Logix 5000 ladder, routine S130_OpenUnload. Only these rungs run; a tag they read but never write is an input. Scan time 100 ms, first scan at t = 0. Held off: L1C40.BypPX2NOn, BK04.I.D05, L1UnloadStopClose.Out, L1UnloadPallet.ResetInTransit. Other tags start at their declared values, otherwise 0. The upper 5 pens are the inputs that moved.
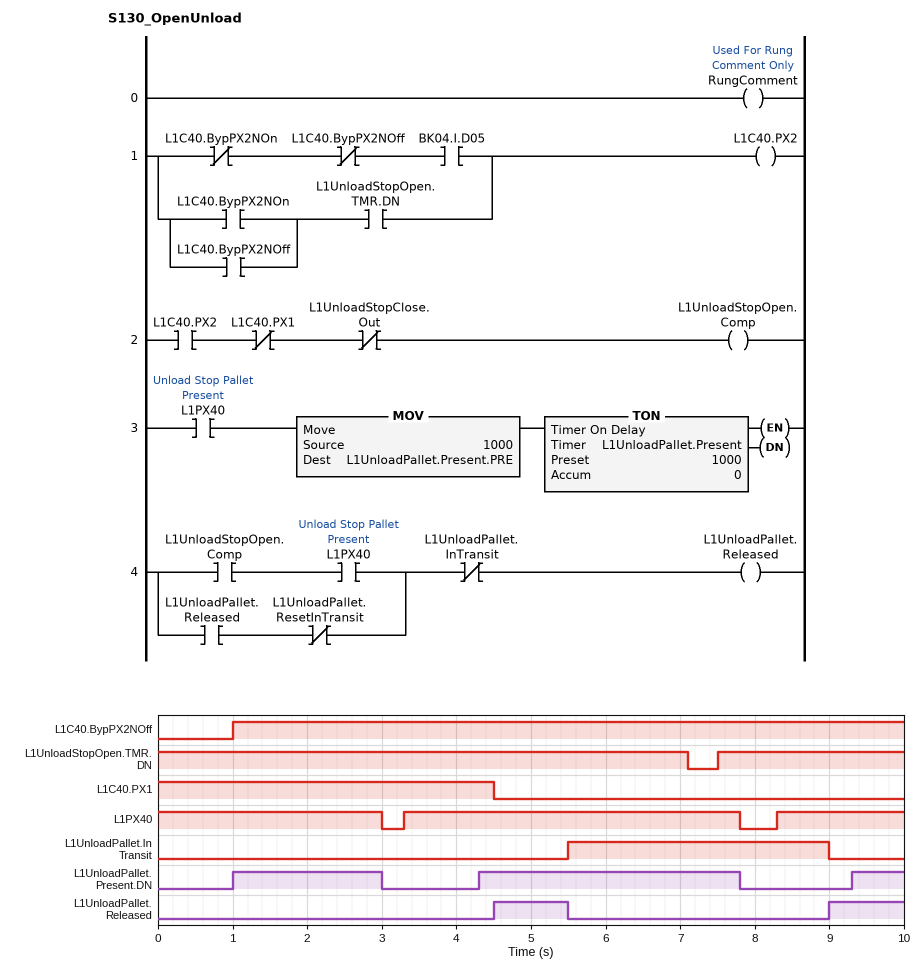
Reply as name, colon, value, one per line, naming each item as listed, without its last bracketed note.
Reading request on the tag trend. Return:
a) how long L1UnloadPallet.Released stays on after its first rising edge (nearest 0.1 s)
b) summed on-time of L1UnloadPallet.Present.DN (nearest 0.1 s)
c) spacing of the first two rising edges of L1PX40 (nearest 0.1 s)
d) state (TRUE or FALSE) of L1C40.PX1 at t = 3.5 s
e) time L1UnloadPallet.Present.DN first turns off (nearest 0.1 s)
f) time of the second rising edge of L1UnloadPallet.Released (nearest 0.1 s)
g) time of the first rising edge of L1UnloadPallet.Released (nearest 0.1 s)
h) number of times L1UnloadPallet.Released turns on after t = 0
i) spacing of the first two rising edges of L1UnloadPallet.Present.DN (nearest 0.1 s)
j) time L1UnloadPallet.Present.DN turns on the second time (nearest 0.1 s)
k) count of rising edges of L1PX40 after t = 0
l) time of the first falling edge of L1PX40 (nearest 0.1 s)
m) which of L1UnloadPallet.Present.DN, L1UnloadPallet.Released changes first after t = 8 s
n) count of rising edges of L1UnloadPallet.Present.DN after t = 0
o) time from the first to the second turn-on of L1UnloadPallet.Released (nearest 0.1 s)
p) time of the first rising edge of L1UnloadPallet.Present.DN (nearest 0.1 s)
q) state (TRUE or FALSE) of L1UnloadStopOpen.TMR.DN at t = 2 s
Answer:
how long L1UnloadPallet.Released stays on after its first rising edge: 1.0 s
summed on-time of L1UnloadPallet.Present.DN: 6.2 s
spacing of the first two rising edges of L1PX40: 5.0 s
state (TRUE or FALSE) of L1C40.PX1 at t = 3.5 s: TRUE
time L1UnloadPallet.Present.DN first turns off: 3.0 s
time of the second rising edge of L1UnloadPallet.Released: 9.0 s
time of the first rising edge of L1UnloadPallet.Released: 4.5 s
number of times L1UnloadPallet.Released turns on after t = 0: 2
spacing of the first two rising edges of L1UnloadPallet.Present.DN: 3.3 s
time L1UnloadPallet.Present.DN turns on the second time: 4.3 s
count of rising edges of L1PX40 after t = 0: 2
time of the first falling edge of L1PX40: 3.0 s
which of L1UnloadPallet.Present.DN, L1UnloadPallet.Released changes first after t = 8 s: L1UnloadPallet.Released
count of rising edges of L1UnloadPallet.Present.DN after t = 0: 3
time from the first to the second turn-on of L1UnloadPallet.Released: 4.5 s
time of the first rising edge of L1UnloadPallet.Present.DN: 1.0 s
state (TRUE or FALSE) of L1UnloadStopOpen.TMR.DN at t = 2 s: TRUE
